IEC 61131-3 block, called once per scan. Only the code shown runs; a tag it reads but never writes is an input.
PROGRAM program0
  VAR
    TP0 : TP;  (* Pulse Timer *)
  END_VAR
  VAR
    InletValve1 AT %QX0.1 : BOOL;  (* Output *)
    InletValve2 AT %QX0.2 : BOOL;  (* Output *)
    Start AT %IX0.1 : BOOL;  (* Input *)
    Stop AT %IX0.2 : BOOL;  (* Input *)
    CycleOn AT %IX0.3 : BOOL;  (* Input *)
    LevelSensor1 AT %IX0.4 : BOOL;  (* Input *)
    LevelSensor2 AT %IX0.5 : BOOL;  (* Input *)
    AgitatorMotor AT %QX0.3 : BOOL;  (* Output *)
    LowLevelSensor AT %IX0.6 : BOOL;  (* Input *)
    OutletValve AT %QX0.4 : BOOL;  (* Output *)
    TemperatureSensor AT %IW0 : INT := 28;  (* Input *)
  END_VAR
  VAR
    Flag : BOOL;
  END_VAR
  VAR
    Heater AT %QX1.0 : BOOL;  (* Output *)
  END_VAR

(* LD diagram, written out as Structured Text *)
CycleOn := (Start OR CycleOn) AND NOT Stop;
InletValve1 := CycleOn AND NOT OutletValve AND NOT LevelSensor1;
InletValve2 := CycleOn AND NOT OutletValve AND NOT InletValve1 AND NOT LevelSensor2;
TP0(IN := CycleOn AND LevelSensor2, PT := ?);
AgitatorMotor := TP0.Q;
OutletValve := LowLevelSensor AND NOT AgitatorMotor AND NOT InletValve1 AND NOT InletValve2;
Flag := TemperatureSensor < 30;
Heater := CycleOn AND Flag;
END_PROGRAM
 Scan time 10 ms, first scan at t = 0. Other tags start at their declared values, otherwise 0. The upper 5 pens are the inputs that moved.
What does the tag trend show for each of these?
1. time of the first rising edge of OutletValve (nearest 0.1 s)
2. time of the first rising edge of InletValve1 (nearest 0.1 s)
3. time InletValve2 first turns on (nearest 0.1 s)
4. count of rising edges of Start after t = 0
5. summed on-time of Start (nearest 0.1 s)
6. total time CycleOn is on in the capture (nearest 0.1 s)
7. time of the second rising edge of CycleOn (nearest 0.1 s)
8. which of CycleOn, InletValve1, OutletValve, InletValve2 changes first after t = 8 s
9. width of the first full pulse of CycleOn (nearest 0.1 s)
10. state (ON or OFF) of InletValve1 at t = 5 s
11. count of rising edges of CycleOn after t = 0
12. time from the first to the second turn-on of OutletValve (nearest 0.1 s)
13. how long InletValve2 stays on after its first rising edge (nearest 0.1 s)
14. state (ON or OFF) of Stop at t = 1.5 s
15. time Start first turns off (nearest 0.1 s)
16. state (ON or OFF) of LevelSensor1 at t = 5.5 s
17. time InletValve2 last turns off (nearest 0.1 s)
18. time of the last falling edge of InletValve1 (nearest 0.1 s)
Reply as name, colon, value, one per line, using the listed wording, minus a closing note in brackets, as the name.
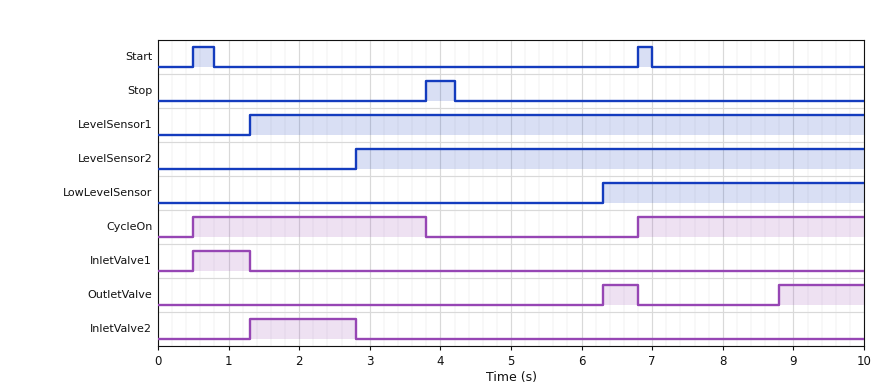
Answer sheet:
time of the first rising edge of OutletValve: 6.3 s
time of the first rising edge of InletValve1: 0.5 s
time InletValve2 first turns on: 1.3 s
count of rising edges of Start after t = 0: 2
summed on-time of Start: 0.5 s
total time CycleOn is on in the capture: 6.5 s
time of the second rising edge of CycleOn: 6.8 s
which of CycleOn, InletValve1, OutletValve, InletValve2 changes first after t = 8 s: OutletValve
width of the first full pulse of CycleOn: 3.3 s
state (ON or OFF) of InletValve1 at t = 5 s: OFF
count of rising edges of CycleOn after t = 0: 2
time from the first to the second turn-on of OutletValve: 2.5 s
how long InletValve2 stays on after its first rising edge: 1.5 s
state (ON or OFF) of Stop at t = 1.5 s: OFF
time Start first turns off: 0.8 s
state (ON or OFF) of LevelSensor1 at t = 5.5 s: ON
time InletValve2 last turns off: 2.8 s
time of the last falling edge of InletValve1: 1.3 s
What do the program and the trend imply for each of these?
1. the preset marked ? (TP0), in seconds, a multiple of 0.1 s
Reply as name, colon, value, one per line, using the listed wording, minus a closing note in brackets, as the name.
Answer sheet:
the preset marked ? (TP0), in seconds, a multiple of 0.1 s: 2.0 s
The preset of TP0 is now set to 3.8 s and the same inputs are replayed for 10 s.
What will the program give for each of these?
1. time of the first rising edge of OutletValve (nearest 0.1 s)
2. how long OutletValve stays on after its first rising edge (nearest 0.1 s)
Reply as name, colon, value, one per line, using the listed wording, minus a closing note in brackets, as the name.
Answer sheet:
time of the first rising edge of OutletValve: 6.6 s
how long OutletValve stays on after its first rising edge: 0.2 s
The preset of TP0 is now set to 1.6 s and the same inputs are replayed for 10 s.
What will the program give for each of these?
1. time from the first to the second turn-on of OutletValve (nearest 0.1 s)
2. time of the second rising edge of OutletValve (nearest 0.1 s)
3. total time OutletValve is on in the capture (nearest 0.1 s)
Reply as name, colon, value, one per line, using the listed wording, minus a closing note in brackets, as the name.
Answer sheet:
time from the first to the second turn-on of OutletValve: 2.1 s
time of the second rising edge of OutletValve: 8.4 s
total time OutletValve is on in the capture: 2.1 s
